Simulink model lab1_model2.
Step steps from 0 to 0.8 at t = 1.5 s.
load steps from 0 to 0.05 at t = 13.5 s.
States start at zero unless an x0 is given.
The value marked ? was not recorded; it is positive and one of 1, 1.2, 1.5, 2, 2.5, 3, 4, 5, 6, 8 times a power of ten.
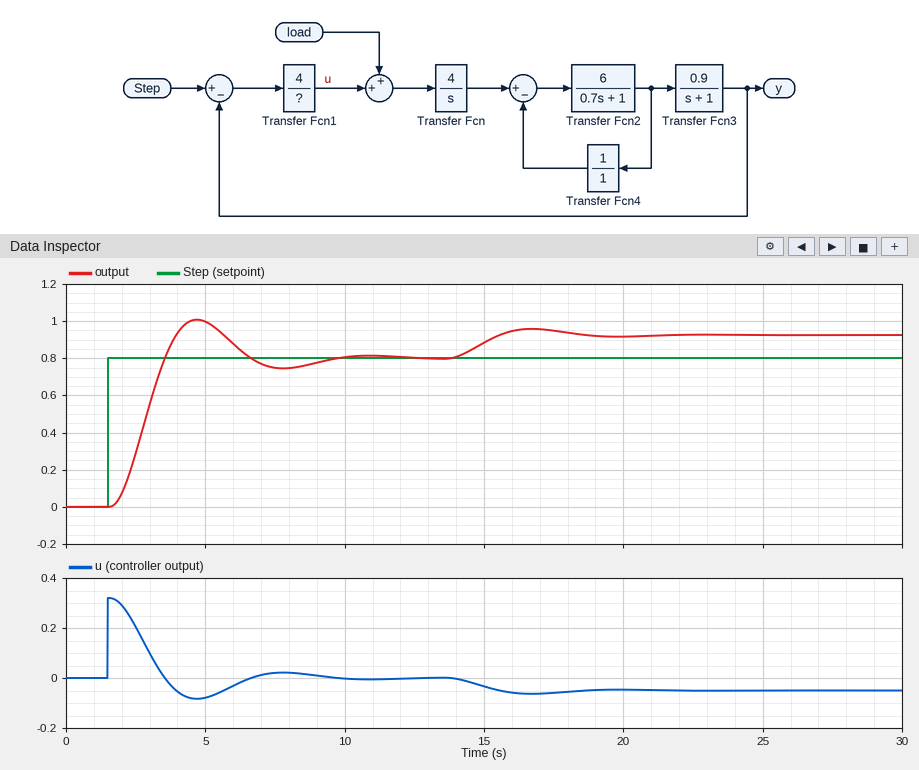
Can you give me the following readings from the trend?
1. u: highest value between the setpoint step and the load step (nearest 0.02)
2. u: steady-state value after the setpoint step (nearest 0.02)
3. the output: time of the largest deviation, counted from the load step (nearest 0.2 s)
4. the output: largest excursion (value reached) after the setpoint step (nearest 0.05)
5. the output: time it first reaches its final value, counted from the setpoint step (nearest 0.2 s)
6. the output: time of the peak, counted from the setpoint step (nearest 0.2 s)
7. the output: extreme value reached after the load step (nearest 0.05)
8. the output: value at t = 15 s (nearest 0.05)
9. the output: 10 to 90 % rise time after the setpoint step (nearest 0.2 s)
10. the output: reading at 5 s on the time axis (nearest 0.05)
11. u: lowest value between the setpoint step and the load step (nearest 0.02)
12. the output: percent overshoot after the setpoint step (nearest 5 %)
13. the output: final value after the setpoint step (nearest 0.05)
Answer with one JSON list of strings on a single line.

["0.32", "0.00", "3.2 s", "1.00", "2.0 s", "3.2 s", "0.95", "0.90", "1.4 s", "1.00", "-0.08", "25 %", "0.80"]
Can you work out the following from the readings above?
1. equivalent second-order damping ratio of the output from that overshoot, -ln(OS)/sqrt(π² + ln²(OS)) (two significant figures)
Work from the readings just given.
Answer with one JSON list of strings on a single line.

["0.40"]
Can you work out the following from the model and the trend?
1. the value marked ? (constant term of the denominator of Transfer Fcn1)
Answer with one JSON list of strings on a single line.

["10"]
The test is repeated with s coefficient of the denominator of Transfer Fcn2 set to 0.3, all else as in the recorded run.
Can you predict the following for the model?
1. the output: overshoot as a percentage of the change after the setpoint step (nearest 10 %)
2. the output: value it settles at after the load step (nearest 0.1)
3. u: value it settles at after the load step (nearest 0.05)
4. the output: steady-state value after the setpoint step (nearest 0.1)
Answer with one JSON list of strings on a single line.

["20 %", "0.9", "-0.05", "0.8"]
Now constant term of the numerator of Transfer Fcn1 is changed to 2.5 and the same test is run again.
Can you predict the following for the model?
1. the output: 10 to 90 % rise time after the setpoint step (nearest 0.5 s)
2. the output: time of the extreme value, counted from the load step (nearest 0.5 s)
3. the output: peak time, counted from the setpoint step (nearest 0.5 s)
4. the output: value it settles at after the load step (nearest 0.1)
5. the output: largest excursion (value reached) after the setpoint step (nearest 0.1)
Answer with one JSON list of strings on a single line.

["2.0 s", "4.5 s", "4.5 s", "1.0", "0.9"]
